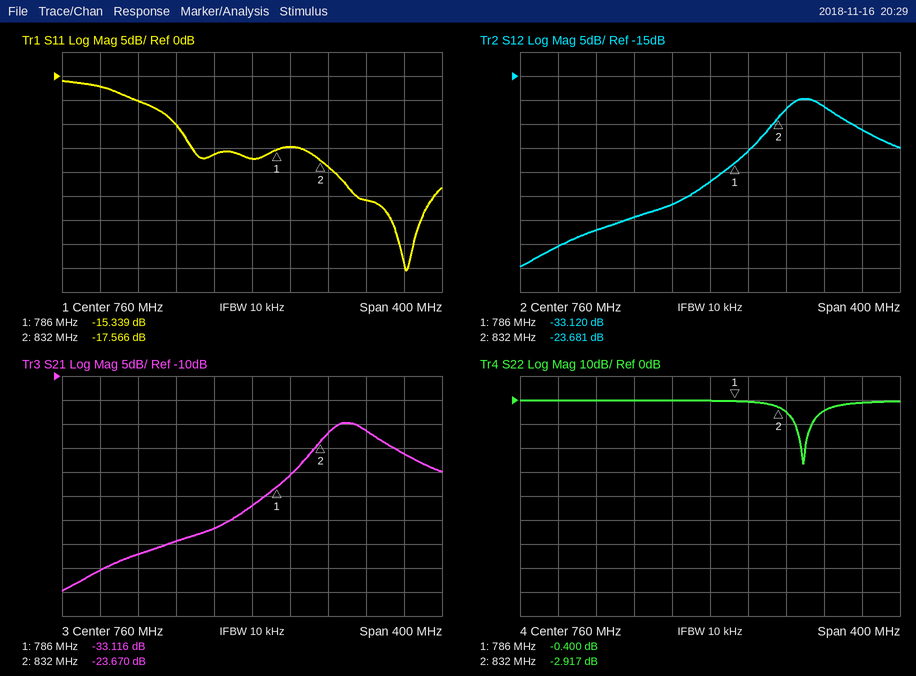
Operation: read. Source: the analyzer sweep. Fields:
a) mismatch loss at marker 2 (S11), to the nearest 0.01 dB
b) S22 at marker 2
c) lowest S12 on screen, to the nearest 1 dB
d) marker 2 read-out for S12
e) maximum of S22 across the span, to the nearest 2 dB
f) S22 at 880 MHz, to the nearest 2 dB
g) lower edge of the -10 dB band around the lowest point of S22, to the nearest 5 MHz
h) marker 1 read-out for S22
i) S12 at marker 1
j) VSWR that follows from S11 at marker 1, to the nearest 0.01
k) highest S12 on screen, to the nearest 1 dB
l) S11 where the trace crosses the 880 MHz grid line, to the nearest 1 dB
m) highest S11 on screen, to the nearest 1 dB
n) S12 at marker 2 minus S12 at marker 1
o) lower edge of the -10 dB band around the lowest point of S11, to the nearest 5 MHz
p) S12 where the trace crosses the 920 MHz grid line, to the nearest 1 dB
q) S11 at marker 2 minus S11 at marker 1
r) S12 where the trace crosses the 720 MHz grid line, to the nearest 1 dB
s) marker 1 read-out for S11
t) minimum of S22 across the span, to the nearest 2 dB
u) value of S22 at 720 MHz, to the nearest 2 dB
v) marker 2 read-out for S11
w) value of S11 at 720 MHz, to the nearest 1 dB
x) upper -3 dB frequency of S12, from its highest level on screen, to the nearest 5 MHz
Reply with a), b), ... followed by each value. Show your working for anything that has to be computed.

a) −10 log10(1 − 10^(-17.566/10)) ≈ 0.08 dB
b) -2.917 dB
c) -55 dB
d) -23.681 dB
e) 0 dB
f) -4 dB
g) 850 MHz
h) -0.400 dB
i) -33.120 dB
j) (1 + 0.1710)/(1 − 0.1710) ≈ 1.41
k) -20 dB
l) -26 dB
m) -1 dB
n) -23.681 − (-33.12) = 9.439 dB
o) 680 MHz
p) -26 dB
q) -17.566 − (-15.339) = -2.227 dB
r) -42 dB
s) -15.339 dB
t) -26 dB
u) 0 dB
v) -17.566 dB
w) -16 dB
x) 890 MHz
